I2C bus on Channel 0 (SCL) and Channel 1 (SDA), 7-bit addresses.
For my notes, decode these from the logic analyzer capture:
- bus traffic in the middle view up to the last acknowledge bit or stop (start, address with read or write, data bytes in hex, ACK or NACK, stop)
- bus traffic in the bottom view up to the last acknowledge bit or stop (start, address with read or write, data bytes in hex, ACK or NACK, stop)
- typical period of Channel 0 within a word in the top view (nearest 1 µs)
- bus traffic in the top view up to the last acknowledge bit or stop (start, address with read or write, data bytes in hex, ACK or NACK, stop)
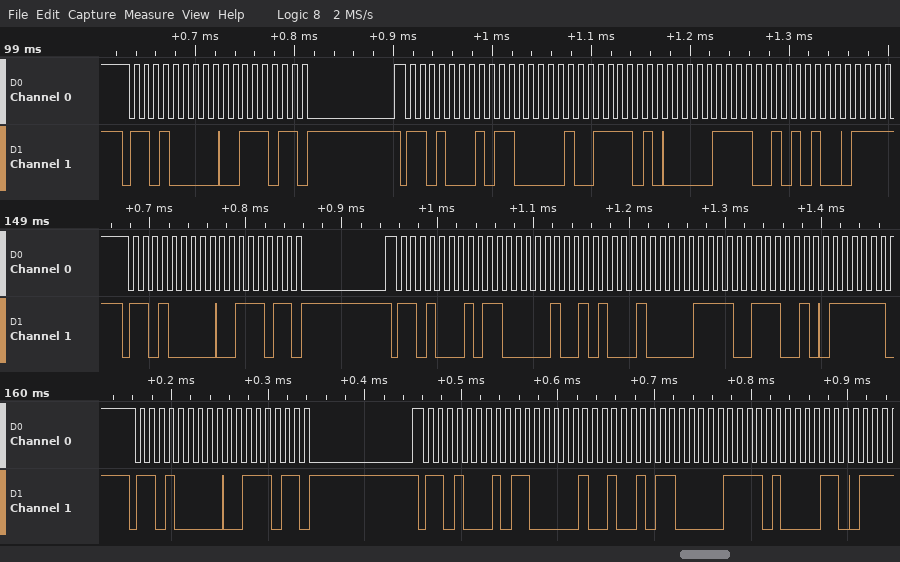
start, address 68 write ACK, 3B ACK, repeated start, address 68 read ACK, C1 ACK, 51 ACK, 0F ACK, 72 ACK
start, address 68 write ACK, 3B ACK, repeated start, address 68 read ACK, C1 ACK, 4B ACK, 0F ACK, 86 ACK
10 µs
start, address 68 write ACK, 3B ACK, repeated start, address 68 read ACK, C1 ACK, 7A ACK, 0F ACK, 54 ACK
